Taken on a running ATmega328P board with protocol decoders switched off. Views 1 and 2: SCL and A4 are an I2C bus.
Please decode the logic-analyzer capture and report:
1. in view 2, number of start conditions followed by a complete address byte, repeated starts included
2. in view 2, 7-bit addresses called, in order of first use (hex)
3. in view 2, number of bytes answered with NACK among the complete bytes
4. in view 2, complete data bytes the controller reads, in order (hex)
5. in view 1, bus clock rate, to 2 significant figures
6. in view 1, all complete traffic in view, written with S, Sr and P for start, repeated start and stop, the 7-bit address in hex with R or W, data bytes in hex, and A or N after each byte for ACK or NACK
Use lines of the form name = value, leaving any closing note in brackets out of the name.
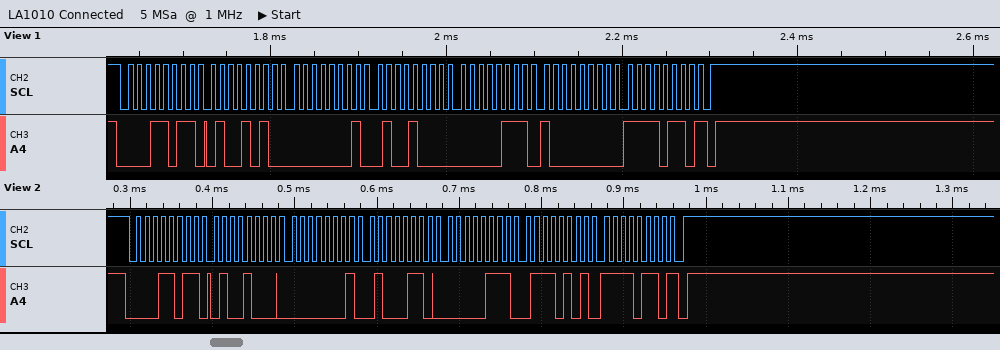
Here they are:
in view 2, number of start conditions followed by a complete address byte, repeated starts included = 1
in view 2, 7-bit addresses called, in order of first use = 0x0D
in view 2, number of bytes answered with NACK among the complete bytes = 1
in view 2, complete data bytes the controller reads, in order = 48 01 46 07 75 F6
in view 1, bus clock rate, to 2 significant figures = 100 kHz
in view 1, all complete traffic in view, written with S, Sr and P for start, repeated start and stop, the 7-bit address in hex with R or W, data bytes in hex, and A or N after each byte for ACK or NACK = S 0DR A 4A A 01 A 48 A 07 A 80 A F6 N P
